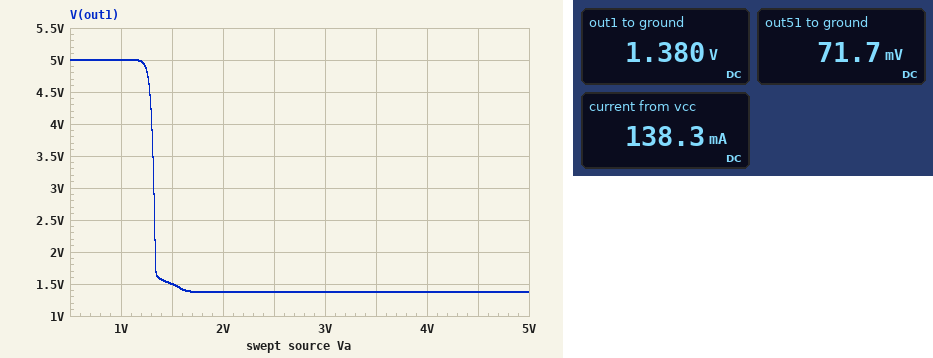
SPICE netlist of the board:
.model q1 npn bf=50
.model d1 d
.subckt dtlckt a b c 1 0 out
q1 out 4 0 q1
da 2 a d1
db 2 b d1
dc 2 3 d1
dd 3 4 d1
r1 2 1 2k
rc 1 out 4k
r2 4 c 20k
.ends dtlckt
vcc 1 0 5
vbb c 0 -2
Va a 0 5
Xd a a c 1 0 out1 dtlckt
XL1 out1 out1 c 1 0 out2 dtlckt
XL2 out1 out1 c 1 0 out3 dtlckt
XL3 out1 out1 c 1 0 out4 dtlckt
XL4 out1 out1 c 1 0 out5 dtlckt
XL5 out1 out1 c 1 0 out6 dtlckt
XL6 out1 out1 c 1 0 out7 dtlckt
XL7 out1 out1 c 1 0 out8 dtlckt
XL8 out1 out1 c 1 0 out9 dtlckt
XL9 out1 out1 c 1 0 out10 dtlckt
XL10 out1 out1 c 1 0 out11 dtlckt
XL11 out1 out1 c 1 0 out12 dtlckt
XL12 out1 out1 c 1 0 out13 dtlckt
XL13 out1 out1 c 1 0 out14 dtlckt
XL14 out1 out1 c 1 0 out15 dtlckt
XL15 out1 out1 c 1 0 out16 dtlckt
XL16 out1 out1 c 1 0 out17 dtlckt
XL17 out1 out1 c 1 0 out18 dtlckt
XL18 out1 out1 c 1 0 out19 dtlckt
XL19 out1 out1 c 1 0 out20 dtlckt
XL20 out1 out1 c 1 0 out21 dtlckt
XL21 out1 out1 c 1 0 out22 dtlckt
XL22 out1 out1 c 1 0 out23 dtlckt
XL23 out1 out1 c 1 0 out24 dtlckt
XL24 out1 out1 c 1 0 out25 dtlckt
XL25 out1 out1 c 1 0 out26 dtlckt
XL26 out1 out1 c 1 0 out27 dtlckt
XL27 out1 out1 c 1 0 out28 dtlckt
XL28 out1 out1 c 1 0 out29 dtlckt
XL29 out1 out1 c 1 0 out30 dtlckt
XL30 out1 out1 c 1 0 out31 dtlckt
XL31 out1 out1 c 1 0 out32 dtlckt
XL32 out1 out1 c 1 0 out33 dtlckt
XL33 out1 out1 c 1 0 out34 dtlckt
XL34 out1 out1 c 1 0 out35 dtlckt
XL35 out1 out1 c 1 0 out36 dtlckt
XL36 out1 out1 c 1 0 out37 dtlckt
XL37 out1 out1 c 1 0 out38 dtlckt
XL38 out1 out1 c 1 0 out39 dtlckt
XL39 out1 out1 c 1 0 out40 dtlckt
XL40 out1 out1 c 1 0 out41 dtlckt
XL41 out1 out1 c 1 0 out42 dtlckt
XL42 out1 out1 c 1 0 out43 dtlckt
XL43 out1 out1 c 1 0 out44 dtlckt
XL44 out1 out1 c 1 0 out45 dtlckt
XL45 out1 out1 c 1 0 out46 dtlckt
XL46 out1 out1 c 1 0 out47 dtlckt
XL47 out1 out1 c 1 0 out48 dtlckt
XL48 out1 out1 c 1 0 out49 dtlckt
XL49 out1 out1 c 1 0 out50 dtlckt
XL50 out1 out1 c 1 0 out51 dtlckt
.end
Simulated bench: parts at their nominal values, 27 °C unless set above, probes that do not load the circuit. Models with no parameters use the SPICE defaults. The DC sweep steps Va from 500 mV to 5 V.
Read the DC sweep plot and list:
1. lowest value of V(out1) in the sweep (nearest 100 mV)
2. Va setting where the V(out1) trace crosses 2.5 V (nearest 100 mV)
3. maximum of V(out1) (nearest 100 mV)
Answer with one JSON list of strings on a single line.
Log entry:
["1.4 V", "1.3 V", "5.0 V"]
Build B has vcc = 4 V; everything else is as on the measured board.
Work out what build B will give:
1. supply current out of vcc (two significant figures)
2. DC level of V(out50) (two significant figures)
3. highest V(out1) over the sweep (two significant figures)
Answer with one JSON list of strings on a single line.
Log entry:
["100 mA", "70 mV", "4.0 V"]
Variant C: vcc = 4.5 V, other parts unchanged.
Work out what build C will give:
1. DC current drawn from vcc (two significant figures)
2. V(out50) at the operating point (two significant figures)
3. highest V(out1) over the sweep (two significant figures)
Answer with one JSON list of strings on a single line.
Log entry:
["120 mA", "71 mV", "4.5 V"]
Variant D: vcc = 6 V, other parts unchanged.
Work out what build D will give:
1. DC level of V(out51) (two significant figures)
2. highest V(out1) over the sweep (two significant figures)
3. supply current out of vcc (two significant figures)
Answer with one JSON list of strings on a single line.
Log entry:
["74 mV", "6.0 V", "180 mA"]
